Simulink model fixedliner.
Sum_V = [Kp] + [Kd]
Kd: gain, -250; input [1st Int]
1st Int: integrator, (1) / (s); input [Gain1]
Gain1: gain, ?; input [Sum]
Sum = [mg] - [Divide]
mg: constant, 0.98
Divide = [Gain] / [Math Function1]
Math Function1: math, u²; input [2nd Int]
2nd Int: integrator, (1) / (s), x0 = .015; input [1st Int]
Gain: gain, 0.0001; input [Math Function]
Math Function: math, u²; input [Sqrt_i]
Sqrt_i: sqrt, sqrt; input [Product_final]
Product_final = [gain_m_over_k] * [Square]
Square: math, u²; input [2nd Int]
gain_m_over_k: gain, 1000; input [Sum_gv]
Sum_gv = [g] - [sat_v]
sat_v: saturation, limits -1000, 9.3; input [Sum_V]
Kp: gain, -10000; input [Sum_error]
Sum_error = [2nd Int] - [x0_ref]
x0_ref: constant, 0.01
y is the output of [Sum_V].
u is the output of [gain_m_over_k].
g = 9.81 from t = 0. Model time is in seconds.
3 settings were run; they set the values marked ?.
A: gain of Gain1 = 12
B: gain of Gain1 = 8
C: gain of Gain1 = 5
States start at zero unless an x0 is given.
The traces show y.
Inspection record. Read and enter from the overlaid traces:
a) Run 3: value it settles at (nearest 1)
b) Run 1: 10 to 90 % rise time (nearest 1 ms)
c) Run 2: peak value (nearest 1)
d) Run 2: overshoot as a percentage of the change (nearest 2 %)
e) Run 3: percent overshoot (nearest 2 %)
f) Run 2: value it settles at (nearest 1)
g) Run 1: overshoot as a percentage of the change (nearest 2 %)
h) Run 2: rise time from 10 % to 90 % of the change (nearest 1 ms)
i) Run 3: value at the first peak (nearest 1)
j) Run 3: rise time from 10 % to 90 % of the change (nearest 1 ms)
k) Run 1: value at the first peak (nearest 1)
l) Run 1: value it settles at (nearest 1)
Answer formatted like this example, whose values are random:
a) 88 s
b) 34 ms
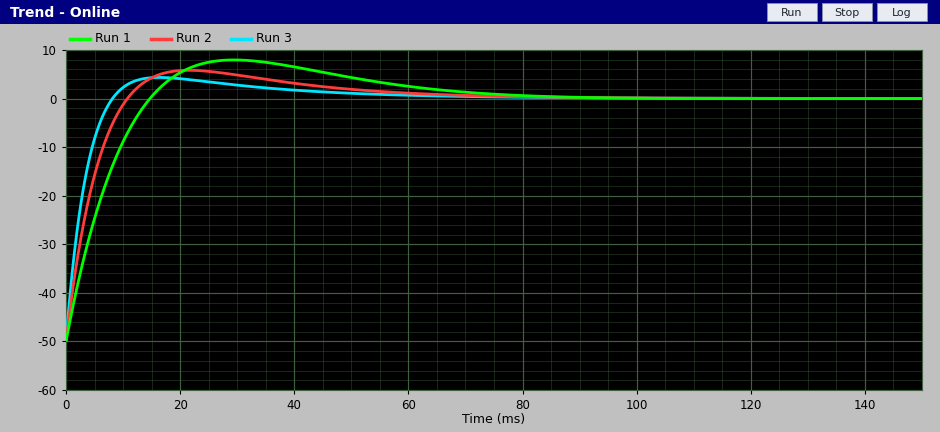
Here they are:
a) 0
b) 11 ms
c) 6
d) 12 %
e) 8 %
f) 0
g) 16 %
h) 8 ms
i) 4
j) 6 ms
k) 8
l) 0
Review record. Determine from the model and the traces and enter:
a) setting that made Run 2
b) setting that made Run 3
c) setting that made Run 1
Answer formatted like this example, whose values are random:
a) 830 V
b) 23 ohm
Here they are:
a) B
b) A
c) C
